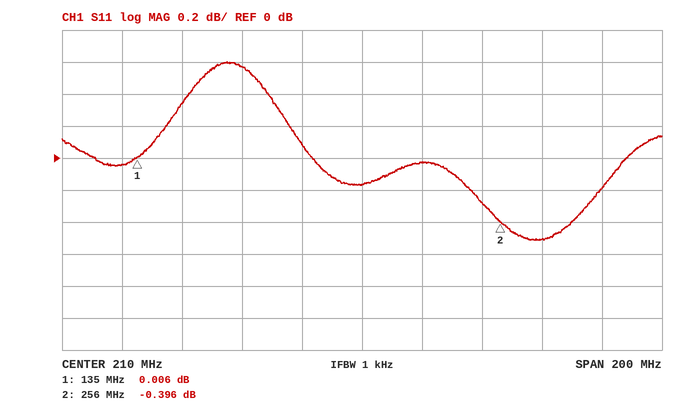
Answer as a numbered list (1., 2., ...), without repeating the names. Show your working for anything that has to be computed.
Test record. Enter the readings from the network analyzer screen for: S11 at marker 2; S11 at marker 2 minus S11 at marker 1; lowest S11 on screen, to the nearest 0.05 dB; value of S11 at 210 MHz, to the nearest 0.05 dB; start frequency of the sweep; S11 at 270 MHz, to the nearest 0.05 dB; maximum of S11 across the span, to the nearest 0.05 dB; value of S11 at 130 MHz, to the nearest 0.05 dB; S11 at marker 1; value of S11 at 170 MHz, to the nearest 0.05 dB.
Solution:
1. -0.396 dB
2. -0.396 − (0.006) = -0.402 dB
3. -0.50 dB
4. -0.15 dB
5. 110 MHz
6. -0.50 dB
7. 0.60 dB
8. -0.05 dB
9. 0.006 dB
10. 0.55 dB
